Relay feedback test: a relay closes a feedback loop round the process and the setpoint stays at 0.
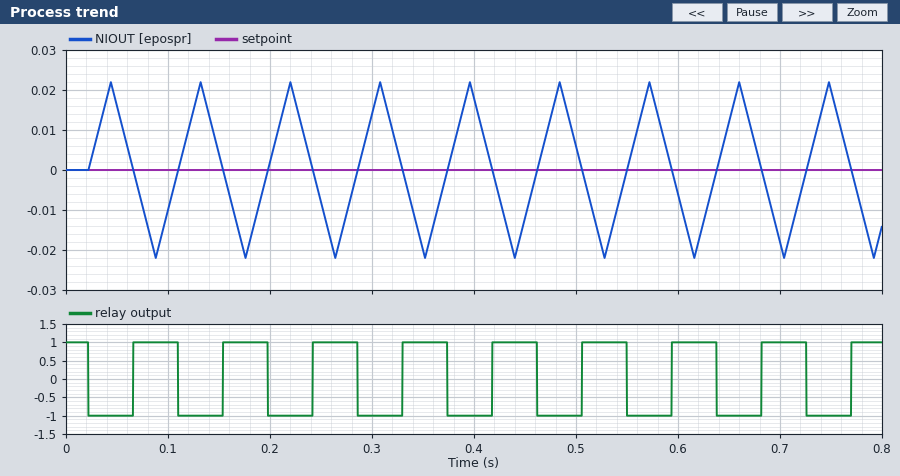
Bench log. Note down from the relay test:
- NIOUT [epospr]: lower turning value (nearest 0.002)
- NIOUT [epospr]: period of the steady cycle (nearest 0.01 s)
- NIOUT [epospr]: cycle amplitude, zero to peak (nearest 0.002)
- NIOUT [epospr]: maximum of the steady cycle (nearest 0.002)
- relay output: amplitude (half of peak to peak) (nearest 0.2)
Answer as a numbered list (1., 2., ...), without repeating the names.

1. -0.022
2. 0.09 s
3. 0.022
4. 0.022
5. 1.0
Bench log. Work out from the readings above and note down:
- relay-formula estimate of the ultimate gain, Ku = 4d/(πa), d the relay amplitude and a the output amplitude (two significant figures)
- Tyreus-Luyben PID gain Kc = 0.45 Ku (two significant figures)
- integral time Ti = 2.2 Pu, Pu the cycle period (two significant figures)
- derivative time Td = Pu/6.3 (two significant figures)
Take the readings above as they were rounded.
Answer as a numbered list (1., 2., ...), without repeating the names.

1. 58
2. 26
3. 0.20 s
4. 0.014 s
